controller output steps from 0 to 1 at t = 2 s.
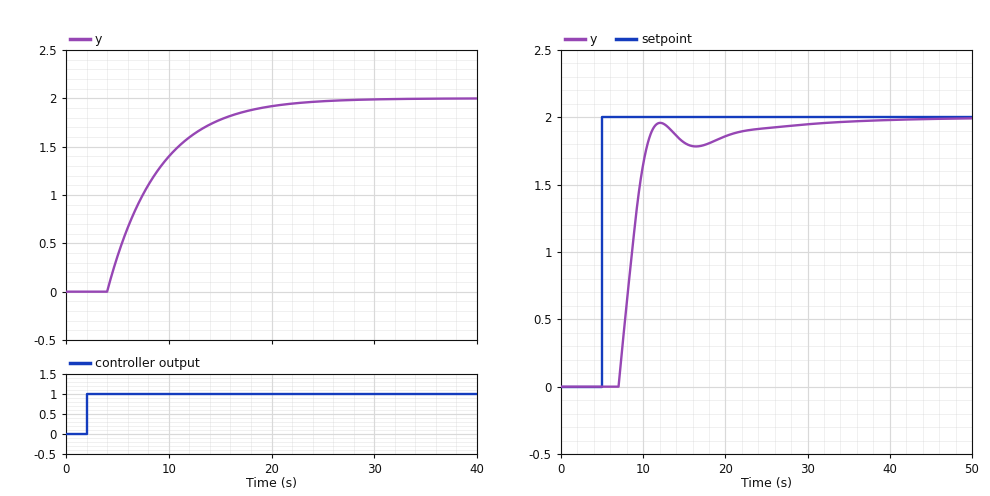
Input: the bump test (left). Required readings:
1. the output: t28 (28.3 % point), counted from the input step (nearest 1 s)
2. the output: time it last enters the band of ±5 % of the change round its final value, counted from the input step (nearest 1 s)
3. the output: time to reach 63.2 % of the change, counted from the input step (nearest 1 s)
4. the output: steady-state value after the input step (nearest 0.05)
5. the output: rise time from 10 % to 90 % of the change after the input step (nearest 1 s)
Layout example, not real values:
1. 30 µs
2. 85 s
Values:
1. 4 s
2. 17 s
3. 7 s
4. 2.00
5. 11 s
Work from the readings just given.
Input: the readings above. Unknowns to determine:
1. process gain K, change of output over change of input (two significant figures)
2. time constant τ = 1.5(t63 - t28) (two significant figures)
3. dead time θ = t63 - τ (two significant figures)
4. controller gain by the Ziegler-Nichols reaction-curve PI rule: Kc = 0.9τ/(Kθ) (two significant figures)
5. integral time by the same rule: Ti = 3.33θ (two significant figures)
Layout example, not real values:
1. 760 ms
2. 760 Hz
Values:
1. 2.0
2. 4.5 s
3. 2.5 s
4. 0.81
5. 8.3 s
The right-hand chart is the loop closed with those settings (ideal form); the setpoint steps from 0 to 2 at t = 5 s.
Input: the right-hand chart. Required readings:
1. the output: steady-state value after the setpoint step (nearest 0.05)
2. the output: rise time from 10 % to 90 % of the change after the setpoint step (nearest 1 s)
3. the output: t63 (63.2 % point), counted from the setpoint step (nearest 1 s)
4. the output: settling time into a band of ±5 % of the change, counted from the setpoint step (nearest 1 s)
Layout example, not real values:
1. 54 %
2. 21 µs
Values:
1. 2.00
2. 3 s
3. 4 s
4. 17 s
